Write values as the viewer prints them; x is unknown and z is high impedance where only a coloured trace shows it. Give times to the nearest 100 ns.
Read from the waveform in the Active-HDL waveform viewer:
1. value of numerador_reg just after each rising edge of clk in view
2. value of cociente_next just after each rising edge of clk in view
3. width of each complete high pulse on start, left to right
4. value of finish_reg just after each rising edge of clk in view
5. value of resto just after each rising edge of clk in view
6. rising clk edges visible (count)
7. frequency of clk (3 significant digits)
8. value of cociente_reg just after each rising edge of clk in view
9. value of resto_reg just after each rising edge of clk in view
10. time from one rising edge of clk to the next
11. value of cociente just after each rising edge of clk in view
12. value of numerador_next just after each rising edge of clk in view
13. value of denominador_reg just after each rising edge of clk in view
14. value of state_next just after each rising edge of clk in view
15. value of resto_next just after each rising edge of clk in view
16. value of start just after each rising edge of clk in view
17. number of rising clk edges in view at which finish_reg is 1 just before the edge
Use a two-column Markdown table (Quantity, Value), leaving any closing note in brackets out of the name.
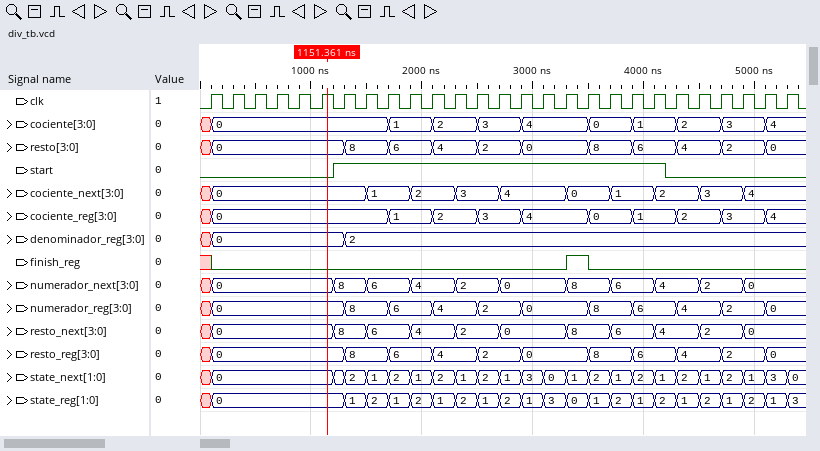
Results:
| Quantity | Value |
|---|---|
| value of numerador_reg just after each rising edge of clk in view | 0, 0, 0, 0, 0, 0, 8, 8, 6, 6, 4, 4, 2, 2, 0, 0, 0, 8, 8, 6, 6, 4, 4, 2, 2, 0, 0 |
| value of cociente_next just after each rising edge of clk in view | 0, 0, 0, 0, 0, 0, 0, 1, 1, 2, 2, 3, 3, 4, 4, 4, 0, 0, 1, 1, 2, 2, 3, 3, 4, 4, 4 |
| width of each complete high pulse on start, left to right | 3000 ns |
| value of finish_reg just after each rising edge of clk in view | 0 0 0 0 0 0 0 0 0 0 0 0 0 0 0 0 1 0 0 0 0 0 0 0 0 0 0 |
| value of resto just after each rising edge of clk in view | 0, 0, 0, 0, 0, 0, 8, 8, 6, 6, 4, 4, 2, 2, 0, 0, 0, 8, 8, 6, 6, 4, 4, 2, 2, 0, 0 |
| rising clk edges visible | 27 |
| frequency of clk | 5.00 MHz |
| value of cociente_reg just after each rising edge of clk in view | 0, 0, 0, 0, 0, 0, 0, 0, 1, 1, 2, 2, 3, 3, 4, 4, 4, 0, 0, 1, 1, 2, 2, 3, 3, 4, 4 |
| value of resto_reg just after each rising edge of clk in view | 0, 0, 0, 0, 0, 0, 8, 8, 6, 6, 4, 4, 2, 2, 0, 0, 0, 8, 8, 6, 6, 4, 4, 2, 2, 0, 0 |
| time from one rising edge of clk to the next | 200 ns |
| value of cociente just after each rising edge of clk in view | 0, 0, 0, 0, 0, 0, 0, 0, 1, 1, 2, 2, 3, 3, 4, 4, 4, 0, 0, 1, 1, 2, 2, 3, 3, 4, 4 |
| value of numerador_next just after each rising edge of clk in view | 0, 0, 0, 0, 0, 0, 8, 6, 6, 4, 4, 2, 2, 0, 0, 0, 8, 8, 6, 6, 4, 4, 2, 2, 0, 0, 0 |
| value of denominador_reg just after each rising edge of clk in view | 0, 0, 0, 0, 0, 0, 2, 2, 2, 2, 2, 2, 2, 2, 2, 2, 2, 2, 2, 2, 2, 2, 2, 2, 2, 2, 2 |
| value of state_next just after each rising edge of clk in view | 0, 0, 0, 0, 0, 0, 2, 1, 2, 1, 2, 1, 2, 1, 3, 0, 1, 2, 1, 2, 1, 2, 1, 2, 1, 3, 0 |
| value of resto_next just after each rising edge of clk in view | 0, 0, 0, 0, 0, 0, 8, 6, 6, 4, 4, 2, 2, 0, 0, 0, 8, 8, 6, 6, 4, 4, 2, 2, 0, 0, 0 |
| value of start just after each rising edge of clk in view | 0 0 0 0 0 0 1 1 1 1 1 1 1 1 1 1 1 1 1 1 1 0 0 0 0 0 0 |
| number of rising clk edges in view at which finish_reg is 1 just before the edge | 1 |
